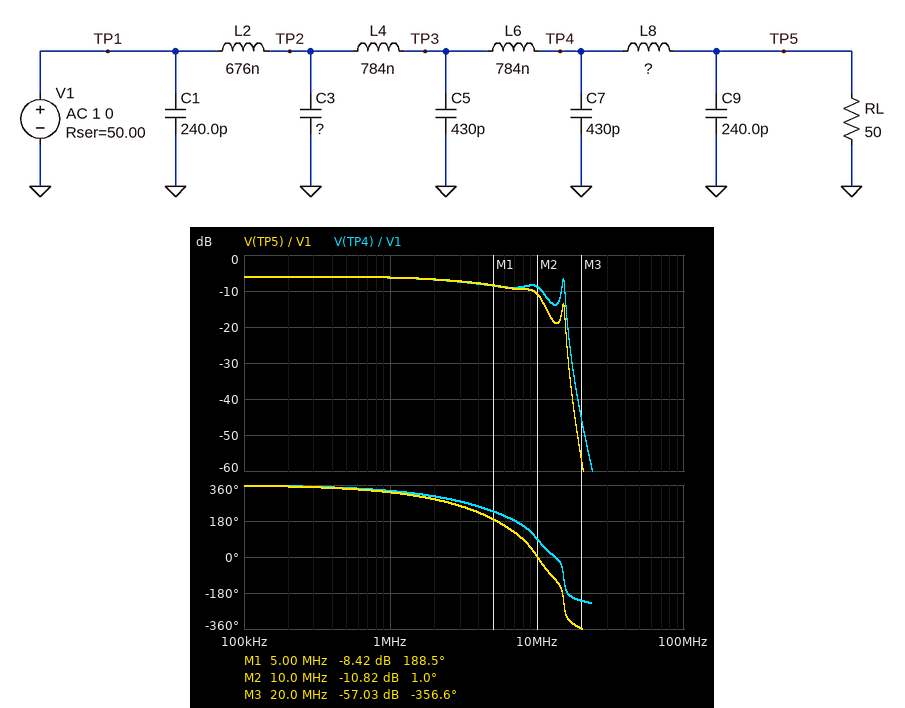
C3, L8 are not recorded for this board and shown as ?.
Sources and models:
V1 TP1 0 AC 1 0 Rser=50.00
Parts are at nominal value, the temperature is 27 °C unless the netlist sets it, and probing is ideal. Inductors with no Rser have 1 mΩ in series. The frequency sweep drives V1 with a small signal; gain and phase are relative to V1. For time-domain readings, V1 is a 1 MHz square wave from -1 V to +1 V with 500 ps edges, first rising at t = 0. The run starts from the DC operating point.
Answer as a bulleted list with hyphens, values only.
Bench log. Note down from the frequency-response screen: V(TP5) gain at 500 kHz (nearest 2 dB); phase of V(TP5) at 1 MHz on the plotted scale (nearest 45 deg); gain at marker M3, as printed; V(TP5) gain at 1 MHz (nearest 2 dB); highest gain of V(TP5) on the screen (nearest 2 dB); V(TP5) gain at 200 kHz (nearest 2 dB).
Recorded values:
- -6 dB
- 315 deg
- -57.03 dB
- -6 dB
- -6 dB
- -6 dB
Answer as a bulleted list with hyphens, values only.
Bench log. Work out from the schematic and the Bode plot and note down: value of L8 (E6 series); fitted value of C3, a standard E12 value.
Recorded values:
- 1 µH
- 1.5 nF
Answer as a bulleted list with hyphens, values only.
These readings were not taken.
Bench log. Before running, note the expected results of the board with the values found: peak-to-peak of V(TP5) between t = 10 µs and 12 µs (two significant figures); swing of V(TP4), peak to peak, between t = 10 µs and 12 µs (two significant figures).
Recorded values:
- 1.0 V
- 1.1 V
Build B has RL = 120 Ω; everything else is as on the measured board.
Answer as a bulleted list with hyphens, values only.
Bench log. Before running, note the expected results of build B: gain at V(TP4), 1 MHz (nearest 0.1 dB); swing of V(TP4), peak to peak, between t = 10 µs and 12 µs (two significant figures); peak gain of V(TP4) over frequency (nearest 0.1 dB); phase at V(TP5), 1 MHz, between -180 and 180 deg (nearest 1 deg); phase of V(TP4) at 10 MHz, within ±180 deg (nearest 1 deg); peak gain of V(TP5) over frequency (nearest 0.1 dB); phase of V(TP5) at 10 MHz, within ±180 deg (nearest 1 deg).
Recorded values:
- -3.9 dB
- 1.4 V
- -3.0 dB
- -40 deg
- 103 deg
- -2.8 dB
- 19 deg
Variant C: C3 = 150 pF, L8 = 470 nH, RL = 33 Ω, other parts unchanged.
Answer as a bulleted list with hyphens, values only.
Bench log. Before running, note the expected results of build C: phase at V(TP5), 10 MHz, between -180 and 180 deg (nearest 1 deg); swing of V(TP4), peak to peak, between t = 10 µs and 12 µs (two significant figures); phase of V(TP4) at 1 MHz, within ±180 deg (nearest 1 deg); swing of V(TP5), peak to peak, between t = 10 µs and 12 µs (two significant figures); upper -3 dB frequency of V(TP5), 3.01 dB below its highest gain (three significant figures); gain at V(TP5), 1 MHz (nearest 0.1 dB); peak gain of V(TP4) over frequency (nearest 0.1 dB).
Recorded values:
- 121 deg
- 1.0 V
- -17 deg
- 1.0 V
- 13.5 MHz
- -8.0 dB
- -7.6 dB
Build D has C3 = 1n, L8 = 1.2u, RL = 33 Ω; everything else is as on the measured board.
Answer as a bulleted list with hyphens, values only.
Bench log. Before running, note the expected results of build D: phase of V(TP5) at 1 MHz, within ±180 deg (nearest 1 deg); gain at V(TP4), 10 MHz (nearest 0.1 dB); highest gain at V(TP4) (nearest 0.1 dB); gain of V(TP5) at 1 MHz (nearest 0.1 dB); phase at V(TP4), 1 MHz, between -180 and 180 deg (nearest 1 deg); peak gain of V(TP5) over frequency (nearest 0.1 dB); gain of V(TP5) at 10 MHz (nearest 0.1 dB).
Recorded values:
- -32 deg
- -3.2 dB
- 2.8 dB
- -7.9 dB
- -19 deg
- -7.8 dB
- -10.4 dB
